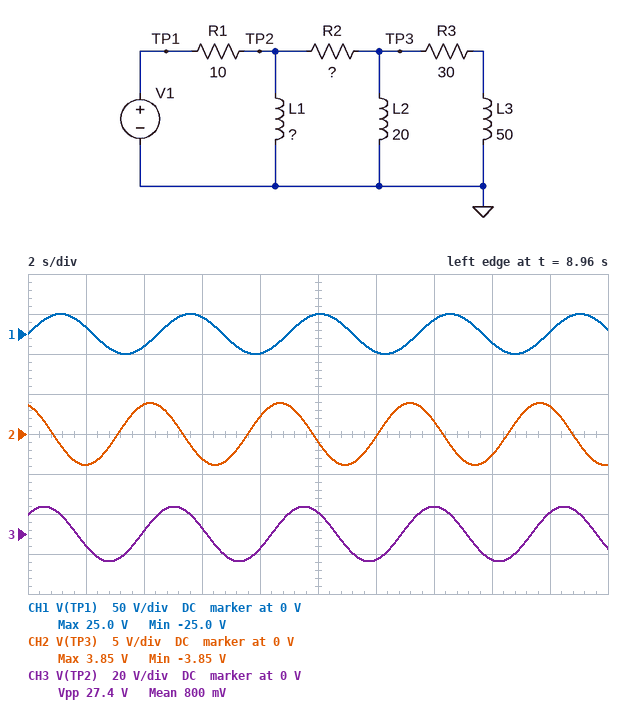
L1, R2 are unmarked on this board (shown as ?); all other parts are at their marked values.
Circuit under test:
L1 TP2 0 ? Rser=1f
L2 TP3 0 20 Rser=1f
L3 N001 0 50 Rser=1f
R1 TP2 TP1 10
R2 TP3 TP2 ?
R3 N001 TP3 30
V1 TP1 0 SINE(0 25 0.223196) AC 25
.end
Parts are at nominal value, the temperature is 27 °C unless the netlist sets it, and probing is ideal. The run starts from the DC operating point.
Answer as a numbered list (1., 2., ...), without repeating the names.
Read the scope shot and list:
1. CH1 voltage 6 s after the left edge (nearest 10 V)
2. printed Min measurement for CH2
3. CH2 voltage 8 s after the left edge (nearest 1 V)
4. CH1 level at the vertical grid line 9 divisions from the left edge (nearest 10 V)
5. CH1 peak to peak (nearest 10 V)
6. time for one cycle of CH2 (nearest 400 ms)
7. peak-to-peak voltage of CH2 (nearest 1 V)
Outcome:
1. 20 V
2. -3.85 V
3. 2 V
4. 0 V
5. 50 V
6. 4.4 s
7. 8 V
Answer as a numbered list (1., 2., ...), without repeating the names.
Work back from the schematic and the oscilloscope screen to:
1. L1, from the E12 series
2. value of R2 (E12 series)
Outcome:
1. 5.6 H
2. 68 Ω
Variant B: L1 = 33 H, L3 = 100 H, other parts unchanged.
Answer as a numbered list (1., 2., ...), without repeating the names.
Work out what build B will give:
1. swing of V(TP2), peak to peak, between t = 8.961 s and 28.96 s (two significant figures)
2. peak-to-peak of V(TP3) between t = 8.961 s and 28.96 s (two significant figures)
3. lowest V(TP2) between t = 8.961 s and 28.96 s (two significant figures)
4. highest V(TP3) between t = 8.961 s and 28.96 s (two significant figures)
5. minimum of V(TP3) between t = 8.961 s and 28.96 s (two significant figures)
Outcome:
1. 43 V
2. 14 V
3. -22 V
4. 6.9 V
5. -6.9 V
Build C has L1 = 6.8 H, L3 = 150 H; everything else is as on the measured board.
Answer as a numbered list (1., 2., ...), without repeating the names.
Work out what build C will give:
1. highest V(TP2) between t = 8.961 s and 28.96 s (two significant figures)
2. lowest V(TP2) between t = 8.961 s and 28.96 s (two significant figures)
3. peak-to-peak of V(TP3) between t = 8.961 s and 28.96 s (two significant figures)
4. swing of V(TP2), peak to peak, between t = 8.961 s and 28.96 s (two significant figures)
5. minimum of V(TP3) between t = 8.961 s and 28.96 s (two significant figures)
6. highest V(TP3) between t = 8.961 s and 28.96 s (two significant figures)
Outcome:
1. 15 V
2. -15 V
3. 10 V
4. 30 V
5. -5.1 V
6. 5.1 V
